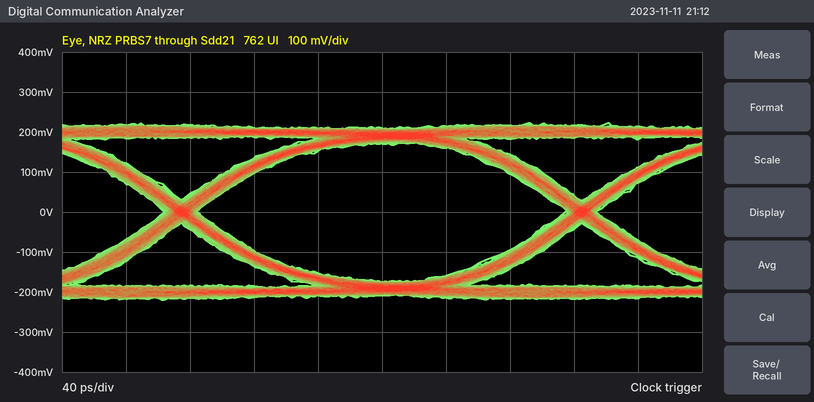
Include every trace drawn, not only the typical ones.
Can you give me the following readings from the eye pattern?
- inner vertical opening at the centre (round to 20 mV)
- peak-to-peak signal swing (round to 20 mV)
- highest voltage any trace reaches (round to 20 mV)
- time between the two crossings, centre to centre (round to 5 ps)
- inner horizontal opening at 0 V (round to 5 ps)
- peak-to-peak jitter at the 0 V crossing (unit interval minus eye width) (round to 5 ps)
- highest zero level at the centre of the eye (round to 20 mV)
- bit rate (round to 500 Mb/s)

340 mV
440 mV
220 mV
250 ps
230 ps
20 ps
-180 mV
4.0 Gb/s
